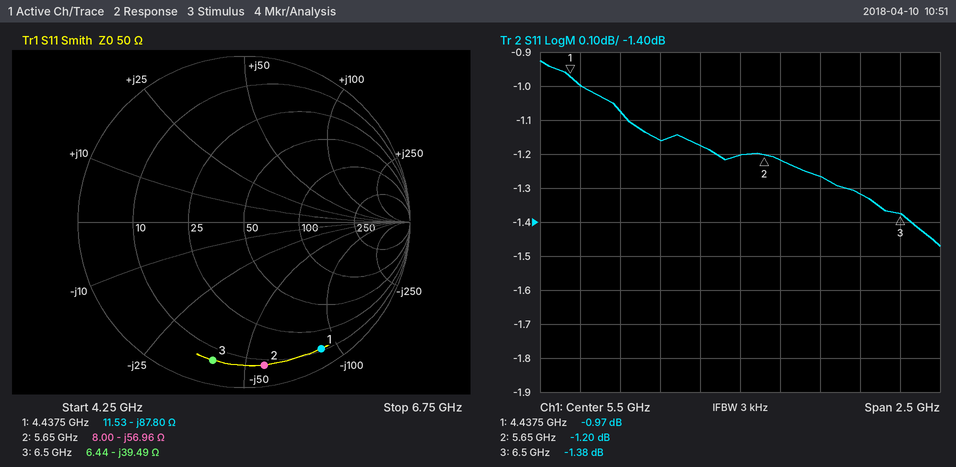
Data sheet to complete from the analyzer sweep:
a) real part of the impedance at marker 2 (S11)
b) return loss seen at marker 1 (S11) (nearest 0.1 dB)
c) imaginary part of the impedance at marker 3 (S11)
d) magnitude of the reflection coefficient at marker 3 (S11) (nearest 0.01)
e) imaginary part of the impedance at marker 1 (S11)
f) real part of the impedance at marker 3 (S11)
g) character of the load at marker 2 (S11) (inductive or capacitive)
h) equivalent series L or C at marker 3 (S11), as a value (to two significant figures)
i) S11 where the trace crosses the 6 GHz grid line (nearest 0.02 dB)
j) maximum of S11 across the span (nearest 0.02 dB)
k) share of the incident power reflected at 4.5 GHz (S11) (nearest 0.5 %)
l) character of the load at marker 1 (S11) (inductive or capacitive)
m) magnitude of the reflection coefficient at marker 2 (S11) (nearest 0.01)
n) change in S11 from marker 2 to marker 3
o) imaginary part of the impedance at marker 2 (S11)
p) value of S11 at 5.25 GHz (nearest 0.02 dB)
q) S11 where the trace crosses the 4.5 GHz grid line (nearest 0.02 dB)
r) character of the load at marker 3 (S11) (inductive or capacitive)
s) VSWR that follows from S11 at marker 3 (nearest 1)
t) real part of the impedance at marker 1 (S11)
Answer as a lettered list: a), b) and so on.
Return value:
a) 8.00 Ω
b) 1.0 dB
c) -39.49 Ω
d) 0.85
e) -87.80 Ω
f) 6.44 Ω
g) capacitive
h) 620 fF
i) -1.26 dB
j) -0.92 dB
k) 79.5 %
l) capacitive
m) 0.87
n) -0.18 dB
o) -56.96 Ω
p) -1.18 dB
q) -1.00 dB
r) capacitive
s) 13
t) 11.53 Ω
